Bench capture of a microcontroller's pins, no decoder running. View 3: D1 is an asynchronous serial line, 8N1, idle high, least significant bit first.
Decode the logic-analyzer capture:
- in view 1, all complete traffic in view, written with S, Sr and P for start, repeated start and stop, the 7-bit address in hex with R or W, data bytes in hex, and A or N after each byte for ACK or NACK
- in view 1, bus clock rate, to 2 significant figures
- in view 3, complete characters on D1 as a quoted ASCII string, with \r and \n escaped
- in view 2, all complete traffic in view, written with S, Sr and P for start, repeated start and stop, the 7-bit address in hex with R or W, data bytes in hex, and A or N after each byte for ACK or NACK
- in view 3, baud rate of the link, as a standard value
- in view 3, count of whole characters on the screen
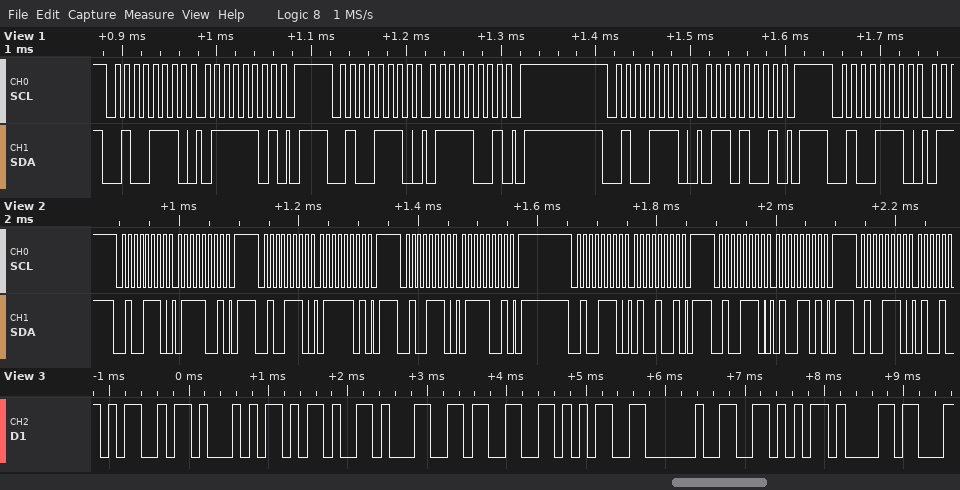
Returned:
S 27W A 7D A P S 27W A 79 A P S 27W A 69 A P S 27W A
100 kHz
"MQ-135 Va"
S 27W A 79 A P S 27W A 7D A P S 27W A 79 A P S 27W A 49 A P S 27W A 4D A P S 27W A
9600 baud
9
